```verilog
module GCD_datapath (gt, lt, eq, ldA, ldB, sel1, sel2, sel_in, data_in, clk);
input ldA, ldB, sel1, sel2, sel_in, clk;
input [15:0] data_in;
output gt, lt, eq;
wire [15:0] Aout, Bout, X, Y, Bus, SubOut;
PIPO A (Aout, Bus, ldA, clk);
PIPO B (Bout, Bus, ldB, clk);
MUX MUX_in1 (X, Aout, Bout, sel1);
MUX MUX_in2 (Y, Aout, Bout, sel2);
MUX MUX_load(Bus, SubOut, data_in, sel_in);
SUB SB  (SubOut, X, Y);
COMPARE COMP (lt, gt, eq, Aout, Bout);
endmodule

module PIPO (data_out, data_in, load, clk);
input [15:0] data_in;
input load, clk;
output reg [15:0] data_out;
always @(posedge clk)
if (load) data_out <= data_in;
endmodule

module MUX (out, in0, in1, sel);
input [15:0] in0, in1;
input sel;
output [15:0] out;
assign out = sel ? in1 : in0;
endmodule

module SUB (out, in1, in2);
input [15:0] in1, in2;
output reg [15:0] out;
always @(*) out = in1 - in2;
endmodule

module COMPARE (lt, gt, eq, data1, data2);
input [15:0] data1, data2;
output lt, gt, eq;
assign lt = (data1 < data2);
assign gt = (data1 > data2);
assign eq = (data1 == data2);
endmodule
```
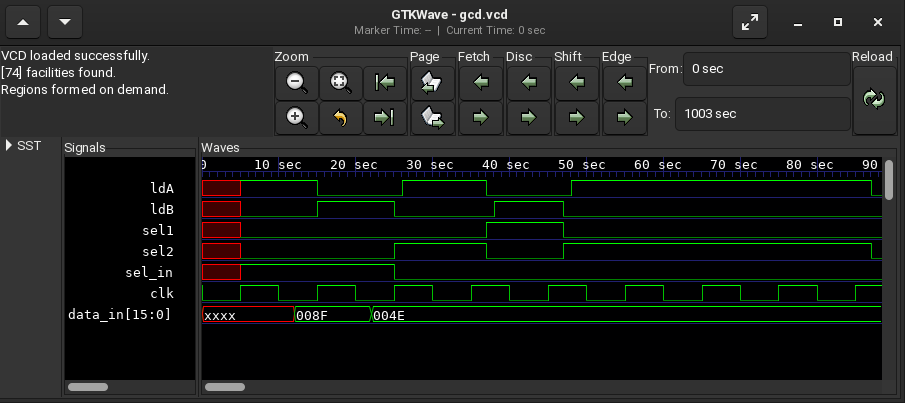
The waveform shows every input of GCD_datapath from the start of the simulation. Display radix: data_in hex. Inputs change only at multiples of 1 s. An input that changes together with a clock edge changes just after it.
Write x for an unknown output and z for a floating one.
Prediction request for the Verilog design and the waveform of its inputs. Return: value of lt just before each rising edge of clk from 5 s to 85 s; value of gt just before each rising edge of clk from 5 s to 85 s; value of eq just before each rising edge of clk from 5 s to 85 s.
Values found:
x x x 0 1 0 0 0 0
x x x 1 0 1 1 1 1
x x x 0 0 0 0 0 0
